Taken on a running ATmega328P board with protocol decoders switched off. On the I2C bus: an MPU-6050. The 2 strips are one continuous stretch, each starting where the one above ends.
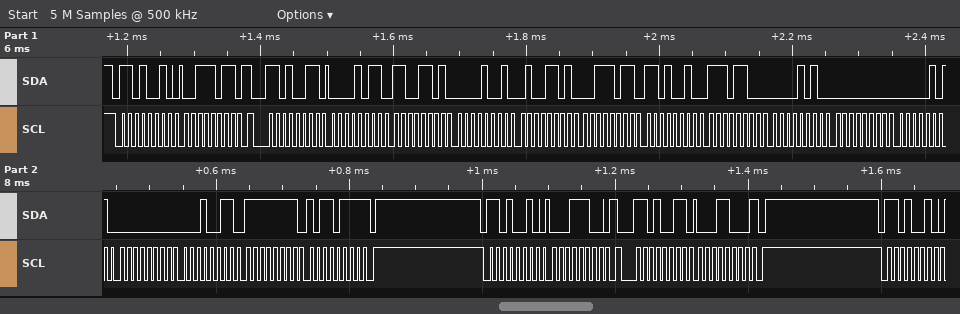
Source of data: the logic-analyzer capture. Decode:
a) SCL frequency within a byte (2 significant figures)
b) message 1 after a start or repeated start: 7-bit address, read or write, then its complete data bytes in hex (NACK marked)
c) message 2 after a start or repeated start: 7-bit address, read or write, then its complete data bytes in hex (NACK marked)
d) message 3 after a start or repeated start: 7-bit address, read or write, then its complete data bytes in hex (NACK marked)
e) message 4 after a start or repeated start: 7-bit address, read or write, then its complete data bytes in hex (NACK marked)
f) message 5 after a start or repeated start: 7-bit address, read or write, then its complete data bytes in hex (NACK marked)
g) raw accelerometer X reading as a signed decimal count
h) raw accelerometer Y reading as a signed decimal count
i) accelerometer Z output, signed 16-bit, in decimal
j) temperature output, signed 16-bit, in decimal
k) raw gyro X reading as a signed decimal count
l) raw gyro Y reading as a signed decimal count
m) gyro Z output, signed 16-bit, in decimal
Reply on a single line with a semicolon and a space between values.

100 kHz; 0x69 write: 3B; 0x69 read: 0B CD 09 4D 3B D2 EC 0A 00 05 00 13 FF B7 NACK; 0x69 write: 1C; 0x69 read: 18 NACK; 0x69 write; 3021; 2381; 15314; -5110; 5; 19; -73
